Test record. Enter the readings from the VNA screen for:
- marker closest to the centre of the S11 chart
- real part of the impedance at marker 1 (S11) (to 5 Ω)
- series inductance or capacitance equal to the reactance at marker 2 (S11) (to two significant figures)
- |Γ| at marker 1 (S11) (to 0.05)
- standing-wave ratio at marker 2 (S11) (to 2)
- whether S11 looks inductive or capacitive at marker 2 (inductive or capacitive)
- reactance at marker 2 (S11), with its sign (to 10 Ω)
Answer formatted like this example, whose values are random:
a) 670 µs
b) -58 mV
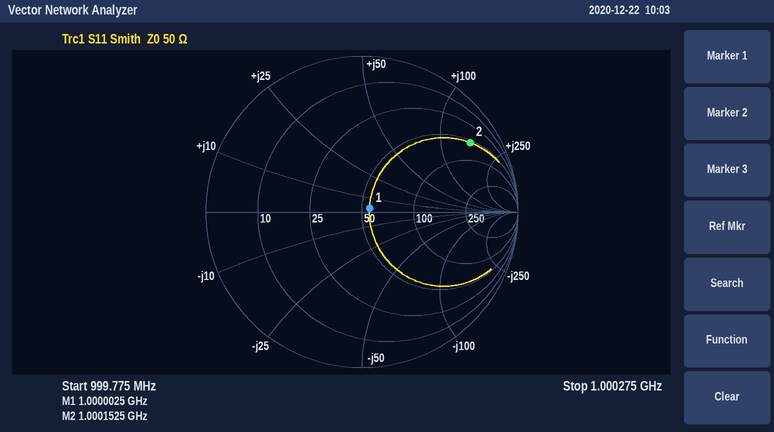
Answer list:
a) marker 1
b) 55 Ω
c) 24 nH
d) 0.05
e) 10
f) inductive
g) +150 Ω
